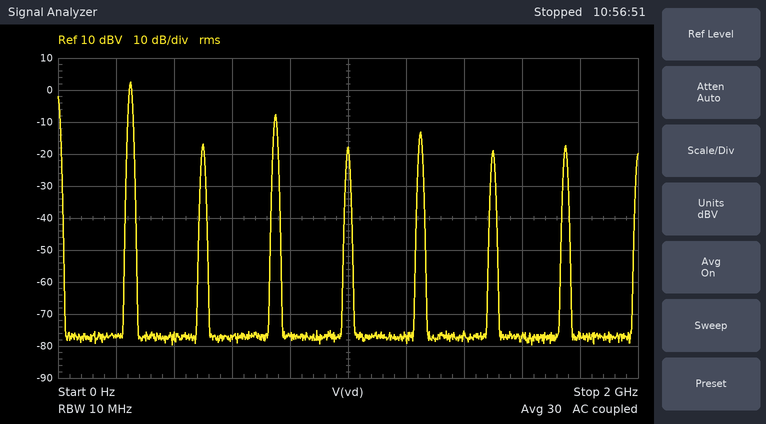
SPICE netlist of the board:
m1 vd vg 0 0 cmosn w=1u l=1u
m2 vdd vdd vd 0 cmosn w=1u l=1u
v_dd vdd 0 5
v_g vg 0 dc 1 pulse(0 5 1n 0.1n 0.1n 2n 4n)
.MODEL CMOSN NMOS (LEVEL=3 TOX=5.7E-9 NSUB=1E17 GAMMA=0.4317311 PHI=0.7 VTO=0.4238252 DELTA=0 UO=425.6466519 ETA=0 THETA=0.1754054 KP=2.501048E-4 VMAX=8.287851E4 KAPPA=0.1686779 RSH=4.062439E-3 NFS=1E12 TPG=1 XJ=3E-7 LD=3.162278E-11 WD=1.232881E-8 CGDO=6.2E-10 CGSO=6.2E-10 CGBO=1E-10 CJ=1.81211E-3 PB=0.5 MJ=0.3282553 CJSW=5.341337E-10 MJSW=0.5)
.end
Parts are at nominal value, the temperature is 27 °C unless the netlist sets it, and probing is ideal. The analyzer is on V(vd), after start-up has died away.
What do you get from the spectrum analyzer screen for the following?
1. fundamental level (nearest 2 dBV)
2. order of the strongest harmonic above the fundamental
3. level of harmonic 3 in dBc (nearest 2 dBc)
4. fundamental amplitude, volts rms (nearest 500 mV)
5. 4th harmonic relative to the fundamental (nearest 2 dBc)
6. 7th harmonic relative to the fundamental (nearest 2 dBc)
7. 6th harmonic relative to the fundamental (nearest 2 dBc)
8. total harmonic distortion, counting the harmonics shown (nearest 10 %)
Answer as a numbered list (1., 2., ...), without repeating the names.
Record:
1. 2 dBV
2. 3
3. -10 dBc
4. 1.5 V
5. -20 dBc
6. -20 dBc
7. -22 dBc
8. 40 %
